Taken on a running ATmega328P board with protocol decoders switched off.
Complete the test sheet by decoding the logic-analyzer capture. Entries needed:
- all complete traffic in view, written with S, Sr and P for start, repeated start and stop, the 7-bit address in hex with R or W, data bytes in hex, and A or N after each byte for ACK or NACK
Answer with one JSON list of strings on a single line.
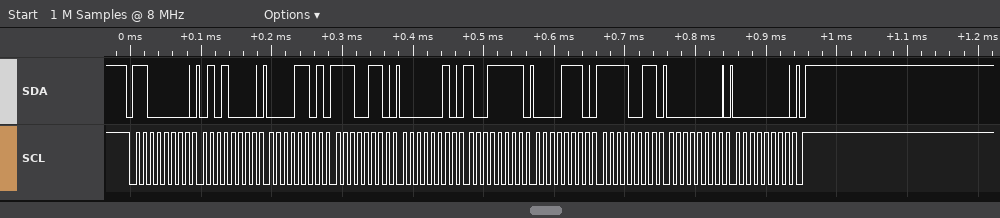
["S 60W A 50 A 0D A E6 A 02 A 9F A 0E A F3 A 00 A 00 A P"]
